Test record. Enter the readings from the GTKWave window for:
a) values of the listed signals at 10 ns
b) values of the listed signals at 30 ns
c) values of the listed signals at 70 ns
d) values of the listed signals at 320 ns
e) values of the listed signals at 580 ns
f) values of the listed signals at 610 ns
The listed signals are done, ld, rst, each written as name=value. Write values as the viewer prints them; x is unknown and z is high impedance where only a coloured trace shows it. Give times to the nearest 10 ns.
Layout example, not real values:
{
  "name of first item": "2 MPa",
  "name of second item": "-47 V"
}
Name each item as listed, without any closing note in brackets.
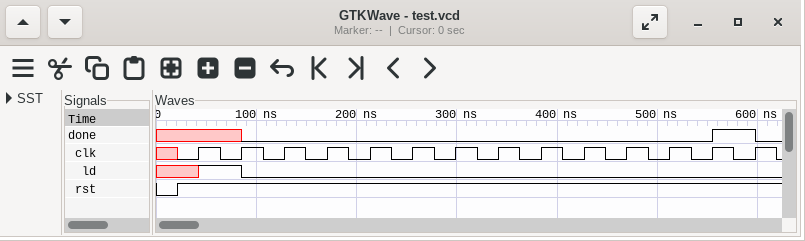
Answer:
{
  "values of the listed signals at 10 ns": "done=x, ld=x, rst=0",
  "values of the listed signals at 30 ns": "done=x, ld=x, rst=1",
  "values of the listed signals at 70 ns": "done=x, ld=1, rst=1",
  "values of the listed signals at 320 ns": "done=0, ld=0, rst=1",
  "values of the listed signals at 580 ns": "done=1, ld=0, rst=1",
  "values of the listed signals at 610 ns": "done=0, ld=0, rst=1"
}
